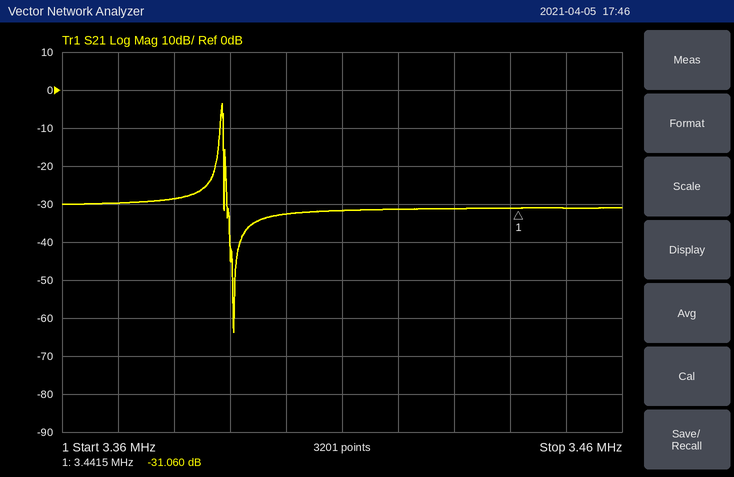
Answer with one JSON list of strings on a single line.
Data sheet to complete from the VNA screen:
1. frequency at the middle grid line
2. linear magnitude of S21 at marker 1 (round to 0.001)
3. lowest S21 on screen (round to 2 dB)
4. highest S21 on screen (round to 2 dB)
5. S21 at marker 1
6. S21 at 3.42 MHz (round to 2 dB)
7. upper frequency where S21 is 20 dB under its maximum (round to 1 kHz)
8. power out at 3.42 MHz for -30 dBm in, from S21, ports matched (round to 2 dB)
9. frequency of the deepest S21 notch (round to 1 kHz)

["3.41 MHz", "0.028", "-64 dB", "-4 dB", "-31.060 dB", "-32 dB", "3.389 MHz", "-62 dBm", "3.391 MHz"]
